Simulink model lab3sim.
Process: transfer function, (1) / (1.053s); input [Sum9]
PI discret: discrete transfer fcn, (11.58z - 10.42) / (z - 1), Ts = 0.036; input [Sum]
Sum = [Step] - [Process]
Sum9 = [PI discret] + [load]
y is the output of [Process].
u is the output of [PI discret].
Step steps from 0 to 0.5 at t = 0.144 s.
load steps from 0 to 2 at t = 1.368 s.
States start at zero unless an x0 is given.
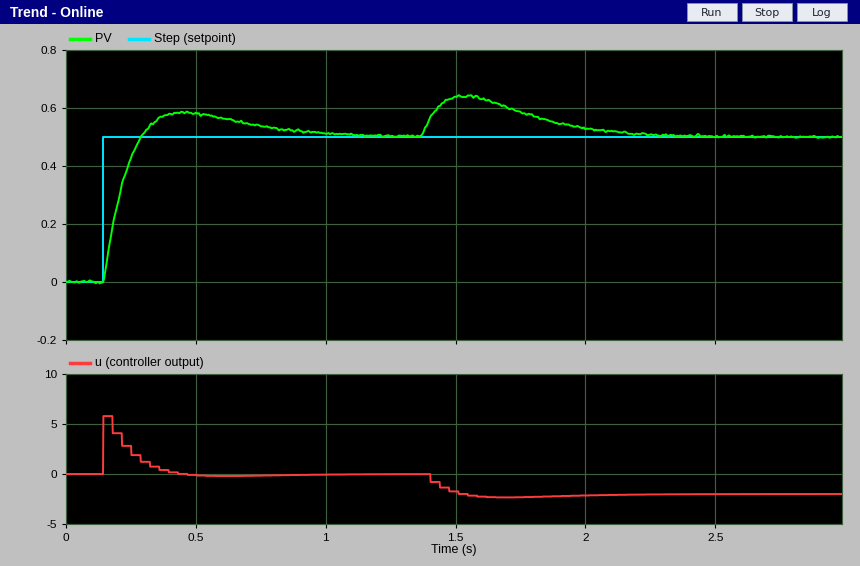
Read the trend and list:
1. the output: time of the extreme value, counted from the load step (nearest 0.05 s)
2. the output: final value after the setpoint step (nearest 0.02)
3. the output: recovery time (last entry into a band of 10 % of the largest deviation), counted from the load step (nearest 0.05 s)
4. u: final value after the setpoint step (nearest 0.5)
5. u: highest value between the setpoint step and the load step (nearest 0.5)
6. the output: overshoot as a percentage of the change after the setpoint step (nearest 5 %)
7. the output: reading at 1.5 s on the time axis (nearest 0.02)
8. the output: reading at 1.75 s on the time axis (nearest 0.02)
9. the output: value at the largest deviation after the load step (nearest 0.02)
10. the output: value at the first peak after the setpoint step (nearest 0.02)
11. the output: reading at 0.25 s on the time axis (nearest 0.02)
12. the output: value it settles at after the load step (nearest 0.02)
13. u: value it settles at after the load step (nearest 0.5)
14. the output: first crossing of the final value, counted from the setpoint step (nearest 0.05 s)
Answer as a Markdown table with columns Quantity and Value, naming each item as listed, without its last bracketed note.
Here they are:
| Quantity | Value |
|---|---|
| the output: time of the extreme value, counted from the load step | 0.20 s |
| the output: final value after the setpoint step | 0.50 |
| the output: recovery time (last entry into a band of 10 % of the largest deviation), counted from the load step | 0.80 s |
| u: final value after the setpoint step | 0.0 |
| u: highest value between the setpoint step and the load step | 6.0 |
| the output: overshoot as a percentage of the change after the setpoint step | 15 % |
| the output: reading at 1.5 s on the time axis | 0.64 |
| the output: reading at 1.75 s on the time axis | 0.58 |
| the output: value at the largest deviation after the load step | 0.64 |
| the output: value at the first peak after the setpoint step | 0.58 |
| the output: reading at 0.25 s on the time axis | 0.42 |
| the output: value it settles at after the load step | 0.50 |
| u: value it settles at after the load step | -2.0 |
| the output: first crossing of the final value, counted from the setpoint step | 0.15 s |
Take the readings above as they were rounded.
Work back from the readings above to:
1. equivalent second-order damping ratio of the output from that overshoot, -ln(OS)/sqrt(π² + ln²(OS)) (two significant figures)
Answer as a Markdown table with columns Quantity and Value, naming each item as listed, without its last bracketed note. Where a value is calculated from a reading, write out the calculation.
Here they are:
| Quantity | Value |
|---|---|
| equivalent second-order damping ratio of the output from that overshoot, -ln(OS)/sqrt(π² + ln²(OS)) | ln(0.15) = -1.897; 1.897 / sqrt(9.870 + 3.599) = 0.52 |
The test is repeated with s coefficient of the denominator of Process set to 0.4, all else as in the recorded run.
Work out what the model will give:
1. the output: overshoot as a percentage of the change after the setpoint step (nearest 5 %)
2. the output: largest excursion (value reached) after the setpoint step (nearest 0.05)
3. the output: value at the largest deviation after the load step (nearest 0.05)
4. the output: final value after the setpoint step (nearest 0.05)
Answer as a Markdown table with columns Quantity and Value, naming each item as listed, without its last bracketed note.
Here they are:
| Quantity | Value |
|---|---|
| the output: overshoot as a percentage of the change after the setpoint step | 10 % |
| the output: largest excursion (value reached) after the setpoint step | 0.55 |
| the output: value at the largest deviation after the load step | 0.70 |
| the output: final value after the setpoint step | 0.50 |
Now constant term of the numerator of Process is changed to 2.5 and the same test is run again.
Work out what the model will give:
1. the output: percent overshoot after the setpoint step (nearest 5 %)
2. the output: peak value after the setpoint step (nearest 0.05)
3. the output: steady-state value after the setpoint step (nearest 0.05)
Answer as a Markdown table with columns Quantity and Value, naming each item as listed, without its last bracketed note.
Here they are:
| Quantity | Value |
|---|---|
| the output: percent overshoot after the setpoint step | 10 % |
| the output: peak value after the setpoint step | 0.55 |
| the output: steady-state value after the setpoint step | 0.50 |
